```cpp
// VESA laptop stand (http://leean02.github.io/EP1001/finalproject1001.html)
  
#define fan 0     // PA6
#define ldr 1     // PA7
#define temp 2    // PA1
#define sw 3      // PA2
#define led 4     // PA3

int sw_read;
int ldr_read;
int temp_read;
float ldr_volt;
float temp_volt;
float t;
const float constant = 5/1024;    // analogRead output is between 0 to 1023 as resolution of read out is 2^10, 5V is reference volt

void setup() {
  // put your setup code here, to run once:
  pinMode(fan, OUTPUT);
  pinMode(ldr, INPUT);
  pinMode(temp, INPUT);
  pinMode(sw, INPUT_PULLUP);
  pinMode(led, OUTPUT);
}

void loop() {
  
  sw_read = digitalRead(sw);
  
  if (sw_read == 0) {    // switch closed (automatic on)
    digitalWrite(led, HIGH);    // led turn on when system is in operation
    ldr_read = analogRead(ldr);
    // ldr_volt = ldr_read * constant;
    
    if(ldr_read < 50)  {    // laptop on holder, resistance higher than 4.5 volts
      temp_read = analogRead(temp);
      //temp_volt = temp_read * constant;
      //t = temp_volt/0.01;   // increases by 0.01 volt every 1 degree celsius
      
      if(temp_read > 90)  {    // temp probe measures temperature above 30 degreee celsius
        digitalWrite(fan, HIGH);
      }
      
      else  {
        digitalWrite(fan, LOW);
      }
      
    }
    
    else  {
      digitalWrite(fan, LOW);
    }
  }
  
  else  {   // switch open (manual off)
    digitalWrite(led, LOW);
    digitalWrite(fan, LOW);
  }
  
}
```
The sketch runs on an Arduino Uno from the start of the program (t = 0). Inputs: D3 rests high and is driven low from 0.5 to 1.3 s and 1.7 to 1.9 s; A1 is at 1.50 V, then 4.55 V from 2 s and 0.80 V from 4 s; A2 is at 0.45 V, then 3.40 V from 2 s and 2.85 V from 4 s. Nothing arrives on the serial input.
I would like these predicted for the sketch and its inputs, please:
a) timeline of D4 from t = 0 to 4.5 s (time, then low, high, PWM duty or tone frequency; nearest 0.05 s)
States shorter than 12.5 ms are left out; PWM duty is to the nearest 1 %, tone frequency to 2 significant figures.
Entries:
0 s low; 0.5 s high; 1.3 s low; 1.7 s high; 1.9 s low
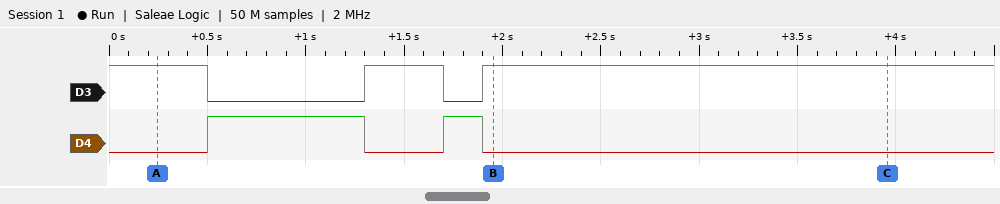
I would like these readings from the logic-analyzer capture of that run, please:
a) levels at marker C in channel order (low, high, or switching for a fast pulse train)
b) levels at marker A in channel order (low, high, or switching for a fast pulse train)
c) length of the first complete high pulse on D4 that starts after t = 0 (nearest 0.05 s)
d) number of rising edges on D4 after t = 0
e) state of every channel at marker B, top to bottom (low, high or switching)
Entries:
D3 high, D4 low
D3 high, D4 low
0.80 s
2
D3 high, D4 low
